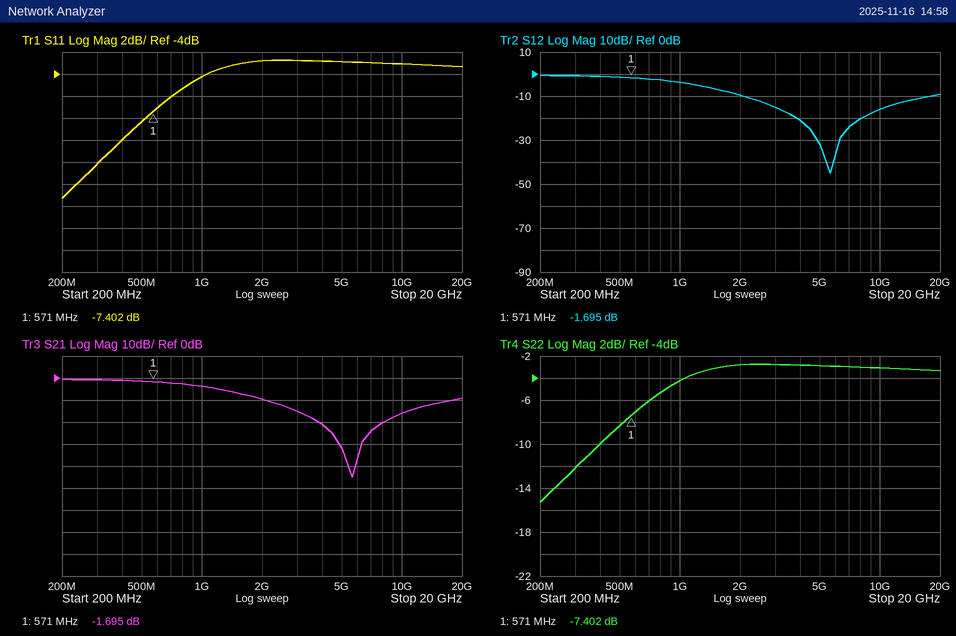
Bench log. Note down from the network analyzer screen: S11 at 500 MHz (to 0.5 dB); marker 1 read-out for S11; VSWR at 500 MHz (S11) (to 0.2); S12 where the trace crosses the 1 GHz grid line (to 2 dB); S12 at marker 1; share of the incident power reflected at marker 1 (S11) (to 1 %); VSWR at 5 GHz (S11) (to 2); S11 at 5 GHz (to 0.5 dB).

-8.5 dB
-7.402 dB
2.2
-4 dB
-1.695 dB
18 %
6
-3.0 dB
